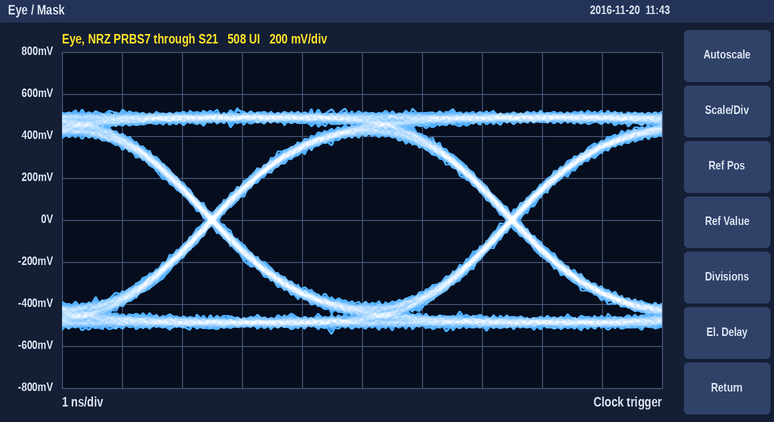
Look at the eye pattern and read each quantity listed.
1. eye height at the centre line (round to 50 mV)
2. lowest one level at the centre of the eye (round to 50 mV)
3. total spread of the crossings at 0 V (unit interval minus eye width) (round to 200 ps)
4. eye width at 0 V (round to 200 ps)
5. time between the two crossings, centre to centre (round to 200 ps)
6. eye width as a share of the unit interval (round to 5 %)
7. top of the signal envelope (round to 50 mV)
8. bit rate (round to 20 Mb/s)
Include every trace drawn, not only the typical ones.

800 mV
400 mV
200 ps
4.8 ns
5.0 ns
95 %
550 mV
200 Mb/s
